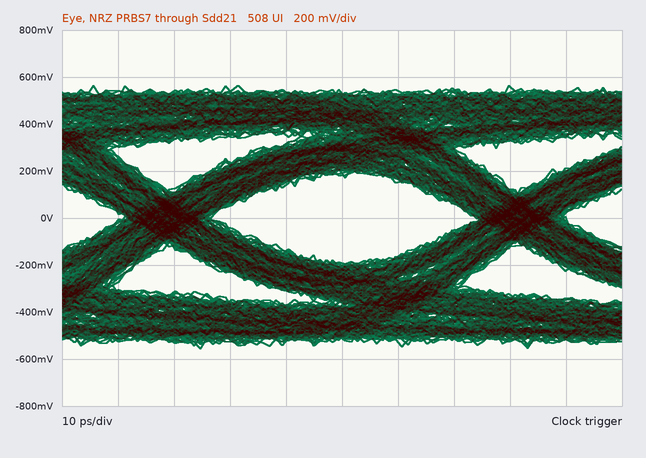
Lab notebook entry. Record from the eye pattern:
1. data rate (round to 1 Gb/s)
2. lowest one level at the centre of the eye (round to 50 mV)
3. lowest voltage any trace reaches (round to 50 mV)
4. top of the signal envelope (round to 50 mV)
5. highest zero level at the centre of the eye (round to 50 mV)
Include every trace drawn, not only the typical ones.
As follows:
16 Gb/s
200 mV
-550 mV
550 mV
-200 mV
